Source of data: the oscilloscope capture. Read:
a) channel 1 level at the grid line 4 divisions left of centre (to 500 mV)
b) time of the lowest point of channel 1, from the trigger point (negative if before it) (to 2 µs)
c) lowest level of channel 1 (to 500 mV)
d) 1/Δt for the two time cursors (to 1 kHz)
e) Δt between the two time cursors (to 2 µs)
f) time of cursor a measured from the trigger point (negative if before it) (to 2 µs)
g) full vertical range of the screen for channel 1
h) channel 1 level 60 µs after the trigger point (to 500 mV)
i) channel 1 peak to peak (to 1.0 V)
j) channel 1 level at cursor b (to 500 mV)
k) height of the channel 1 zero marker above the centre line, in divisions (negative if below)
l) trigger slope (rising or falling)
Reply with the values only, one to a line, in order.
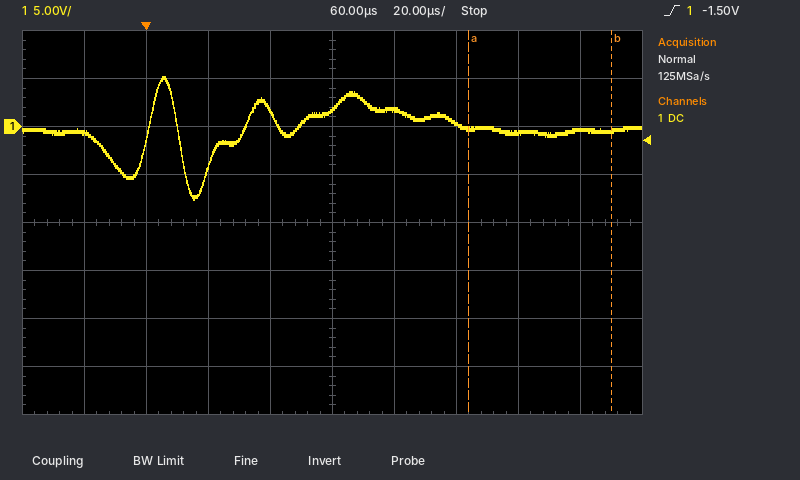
-500 mV
+16 µs
-7.5 V
22 kHz
46 µs
+104 µs
40 V
2.0 V
13.0 V
-500 mV
+2.0 div
rising
